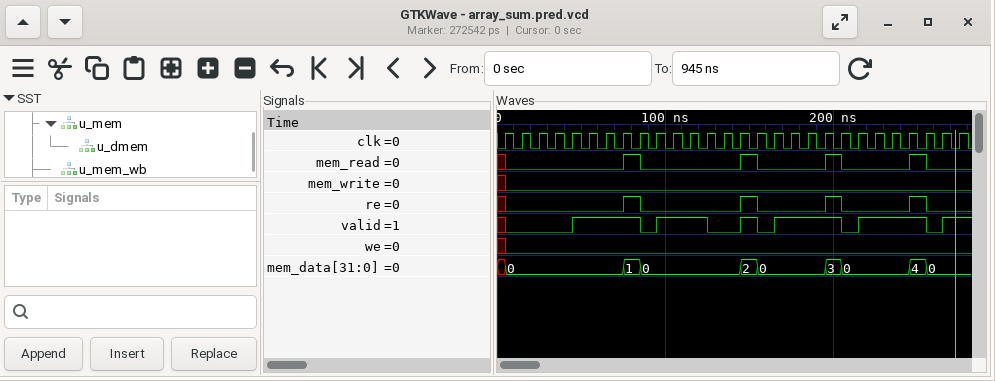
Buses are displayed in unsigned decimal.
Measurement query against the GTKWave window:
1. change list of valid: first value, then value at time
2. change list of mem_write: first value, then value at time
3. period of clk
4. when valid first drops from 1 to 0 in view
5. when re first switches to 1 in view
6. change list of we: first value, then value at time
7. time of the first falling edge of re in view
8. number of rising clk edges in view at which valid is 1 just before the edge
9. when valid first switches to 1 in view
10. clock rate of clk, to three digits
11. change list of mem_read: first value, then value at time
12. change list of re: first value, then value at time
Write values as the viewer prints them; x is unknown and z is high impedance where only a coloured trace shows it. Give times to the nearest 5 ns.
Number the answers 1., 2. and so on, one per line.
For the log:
1. x, 0 at 5 ns, 1 at 45 ns, 0 at 85 ns, 1 at 95 ns, 0 at 125 ns, 1 at 145 ns, 0 at 155 ns, 1 at 165 ns, 0 at 205 ns, 1 at 215 ns, 0 at 255 ns, 1 at 265 ns
2. x, 0 at 5 ns
3. 10 ns
4. 85 ns
5. 75 ns
6. x, 0 at 5 ns
7. 85 ns
8. 17
9. 45 ns
10. 100 MHz
11. x, 0 at 5 ns, 1 at 75 ns, 0 at 85 ns, 1 at 145 ns, 0 at 155 ns, 1 at 195 ns, 0 at 205 ns, 1 at 245 ns, 0 at 255 ns
12. x, 0 at 5 ns, 1 at 75 ns, 0 at 85 ns, 1 at 145 ns, 0 at 155 ns, 1 at 195 ns, 0 at 205 ns, 1 at 245 ns, 0 at 255 ns
